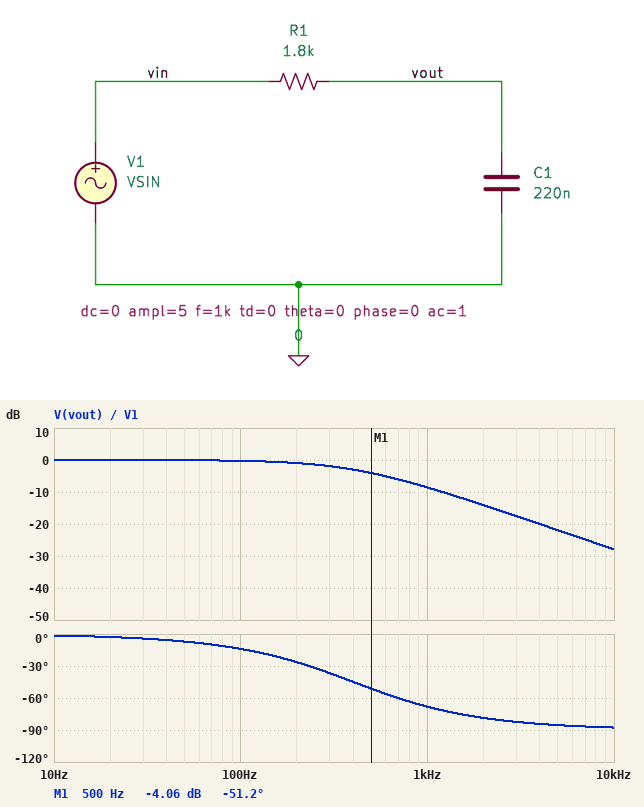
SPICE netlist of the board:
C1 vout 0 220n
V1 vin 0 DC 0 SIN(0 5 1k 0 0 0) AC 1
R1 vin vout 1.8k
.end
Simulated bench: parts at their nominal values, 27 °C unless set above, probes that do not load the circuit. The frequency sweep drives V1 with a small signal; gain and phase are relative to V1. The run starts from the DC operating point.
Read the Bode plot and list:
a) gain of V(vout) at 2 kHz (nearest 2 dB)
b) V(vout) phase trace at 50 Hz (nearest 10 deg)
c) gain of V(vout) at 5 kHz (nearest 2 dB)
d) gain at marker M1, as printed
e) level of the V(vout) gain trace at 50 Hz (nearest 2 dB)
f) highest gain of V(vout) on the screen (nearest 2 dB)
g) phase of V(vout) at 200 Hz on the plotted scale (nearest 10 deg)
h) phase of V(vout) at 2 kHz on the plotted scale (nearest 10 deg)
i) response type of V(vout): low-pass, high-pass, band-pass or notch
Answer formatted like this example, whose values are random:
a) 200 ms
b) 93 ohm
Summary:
a) -14 dB
b) -10 deg
c) -22 dB
d) -4.06 dB
e) 0 dB
f) 0 dB
g) -30 deg
h) -80 deg
i) low-pass
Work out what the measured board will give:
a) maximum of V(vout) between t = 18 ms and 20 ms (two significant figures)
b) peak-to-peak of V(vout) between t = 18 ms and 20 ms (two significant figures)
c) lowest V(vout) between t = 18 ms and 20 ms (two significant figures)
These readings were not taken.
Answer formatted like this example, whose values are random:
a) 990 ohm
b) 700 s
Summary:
a) 1.9 V
b) 3.7 V
c) -1.9 V
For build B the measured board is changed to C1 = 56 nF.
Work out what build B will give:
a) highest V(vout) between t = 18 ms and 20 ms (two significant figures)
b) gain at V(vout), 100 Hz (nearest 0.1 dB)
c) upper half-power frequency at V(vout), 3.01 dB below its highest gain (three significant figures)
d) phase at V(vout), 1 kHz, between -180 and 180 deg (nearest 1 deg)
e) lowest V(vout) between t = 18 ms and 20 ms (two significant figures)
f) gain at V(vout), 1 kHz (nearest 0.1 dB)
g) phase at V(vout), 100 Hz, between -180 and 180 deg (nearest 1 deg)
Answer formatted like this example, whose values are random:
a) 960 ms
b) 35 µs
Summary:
a) 4.2 V
b) 0 dB
c) 1.58 kHz
d) -32 deg
e) -4.2 V
f) -1.5 dB
g) -4 deg
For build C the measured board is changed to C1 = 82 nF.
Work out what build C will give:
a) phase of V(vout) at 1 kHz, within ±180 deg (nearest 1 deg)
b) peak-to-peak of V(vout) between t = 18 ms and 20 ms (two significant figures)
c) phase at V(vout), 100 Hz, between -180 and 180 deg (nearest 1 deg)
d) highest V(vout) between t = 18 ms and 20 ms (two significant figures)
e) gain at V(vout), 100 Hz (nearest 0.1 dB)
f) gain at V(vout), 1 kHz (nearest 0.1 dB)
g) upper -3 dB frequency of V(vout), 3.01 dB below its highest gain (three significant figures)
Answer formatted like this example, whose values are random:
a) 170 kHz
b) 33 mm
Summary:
a) -43 deg
b) 7.3 V
c) -5 deg
d) 3.7 V
e) 0 dB
f) -2.7 dB
g) 1.08 kHz
